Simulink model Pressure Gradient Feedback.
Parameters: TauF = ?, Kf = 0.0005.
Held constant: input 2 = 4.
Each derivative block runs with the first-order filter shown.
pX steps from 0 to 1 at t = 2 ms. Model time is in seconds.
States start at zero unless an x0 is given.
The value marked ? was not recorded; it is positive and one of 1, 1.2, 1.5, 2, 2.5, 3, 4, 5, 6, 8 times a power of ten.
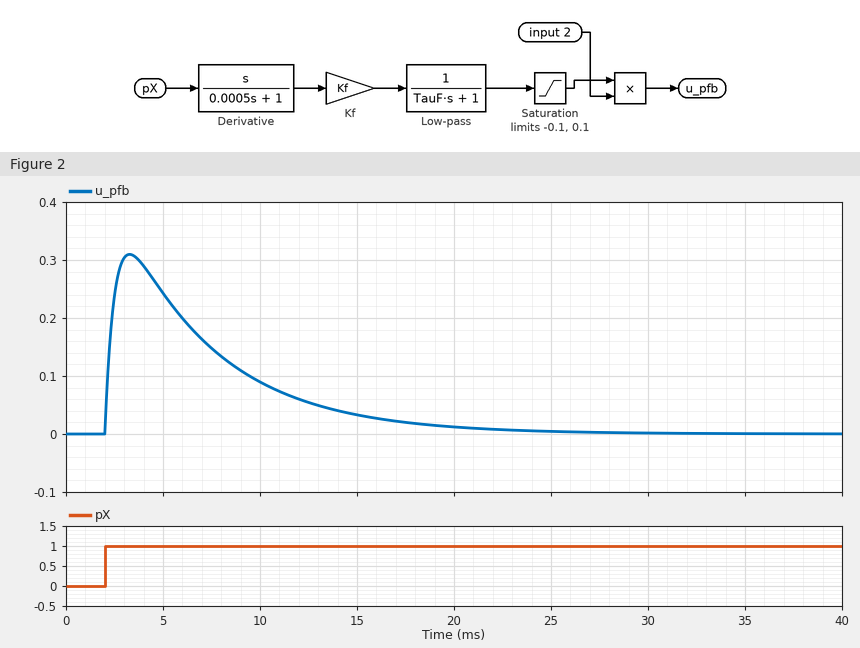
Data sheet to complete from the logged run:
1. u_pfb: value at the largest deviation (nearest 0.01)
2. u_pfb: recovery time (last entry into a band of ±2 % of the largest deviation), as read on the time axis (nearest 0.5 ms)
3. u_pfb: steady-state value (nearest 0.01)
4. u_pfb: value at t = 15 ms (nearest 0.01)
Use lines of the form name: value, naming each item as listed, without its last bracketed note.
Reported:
u_pfb: value at the largest deviation: 0.31
u_pfb: recovery time (last entry into a band of ±2 % of the largest deviation), as read on the time axis: 23.5 ms
u_pfb: steady-state value: 0.00
u_pfb: value at t = 15 ms: 0.03
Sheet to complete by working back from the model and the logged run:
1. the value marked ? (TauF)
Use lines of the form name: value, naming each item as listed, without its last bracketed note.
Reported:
the value marked ?: 0.005
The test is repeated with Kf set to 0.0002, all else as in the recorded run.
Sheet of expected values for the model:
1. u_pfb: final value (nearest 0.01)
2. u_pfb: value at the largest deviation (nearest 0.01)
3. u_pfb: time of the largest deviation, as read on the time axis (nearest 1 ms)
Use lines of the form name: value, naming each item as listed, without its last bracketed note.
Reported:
u_pfb: final value: 0.00
u_pfb: value at the largest deviation: 0.12
u_pfb: time of the largest deviation, as read on the time axis: 3 ms
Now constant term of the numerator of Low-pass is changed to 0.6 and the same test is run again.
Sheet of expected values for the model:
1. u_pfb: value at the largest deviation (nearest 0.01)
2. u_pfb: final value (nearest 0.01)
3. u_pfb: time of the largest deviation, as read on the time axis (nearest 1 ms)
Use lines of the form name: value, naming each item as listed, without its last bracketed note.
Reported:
u_pfb: value at the largest deviation: 0.19
u_pfb: final value: 0.00
u_pfb: time of the largest deviation, as read on the time axis: 3 ms
